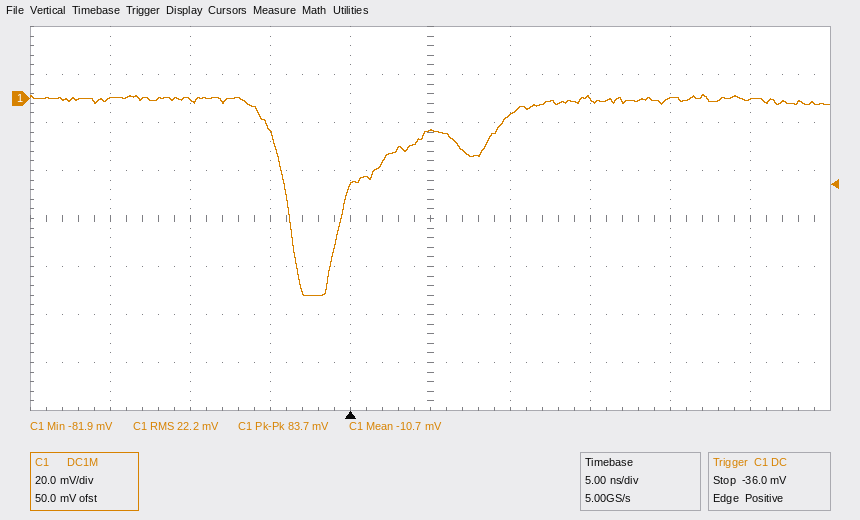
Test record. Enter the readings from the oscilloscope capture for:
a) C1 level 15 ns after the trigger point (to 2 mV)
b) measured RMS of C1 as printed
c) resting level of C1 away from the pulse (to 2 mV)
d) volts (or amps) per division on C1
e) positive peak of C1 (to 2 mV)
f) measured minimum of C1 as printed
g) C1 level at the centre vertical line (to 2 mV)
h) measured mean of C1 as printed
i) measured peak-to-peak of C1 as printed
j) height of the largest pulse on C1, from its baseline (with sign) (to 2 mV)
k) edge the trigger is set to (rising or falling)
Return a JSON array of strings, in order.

["0 mV", "22.2 mV", "0 mV", "20 mV", "2 mV", "-81.9 mV", "-14 mV", "-10.7 mV", "83.7 mV", "-82 mV", "rising"]
